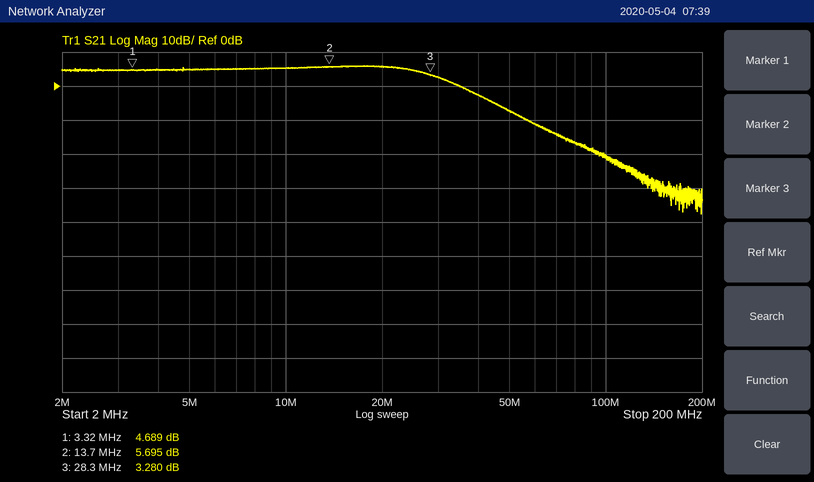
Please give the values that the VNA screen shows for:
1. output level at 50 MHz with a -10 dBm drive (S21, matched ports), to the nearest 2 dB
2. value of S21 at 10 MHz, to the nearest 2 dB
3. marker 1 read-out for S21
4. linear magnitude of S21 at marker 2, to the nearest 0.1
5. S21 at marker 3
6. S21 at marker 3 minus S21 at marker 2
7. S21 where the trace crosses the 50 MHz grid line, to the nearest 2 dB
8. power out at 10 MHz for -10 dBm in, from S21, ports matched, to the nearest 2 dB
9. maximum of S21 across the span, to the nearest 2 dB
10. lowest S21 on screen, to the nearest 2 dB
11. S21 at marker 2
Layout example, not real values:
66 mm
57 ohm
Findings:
-18 dBm
6 dB
4.689 dB
1.9
3.280 dB
-2.415 dB
-8 dB
-4 dBm
6 dB
-38 dB
5.695 dB
